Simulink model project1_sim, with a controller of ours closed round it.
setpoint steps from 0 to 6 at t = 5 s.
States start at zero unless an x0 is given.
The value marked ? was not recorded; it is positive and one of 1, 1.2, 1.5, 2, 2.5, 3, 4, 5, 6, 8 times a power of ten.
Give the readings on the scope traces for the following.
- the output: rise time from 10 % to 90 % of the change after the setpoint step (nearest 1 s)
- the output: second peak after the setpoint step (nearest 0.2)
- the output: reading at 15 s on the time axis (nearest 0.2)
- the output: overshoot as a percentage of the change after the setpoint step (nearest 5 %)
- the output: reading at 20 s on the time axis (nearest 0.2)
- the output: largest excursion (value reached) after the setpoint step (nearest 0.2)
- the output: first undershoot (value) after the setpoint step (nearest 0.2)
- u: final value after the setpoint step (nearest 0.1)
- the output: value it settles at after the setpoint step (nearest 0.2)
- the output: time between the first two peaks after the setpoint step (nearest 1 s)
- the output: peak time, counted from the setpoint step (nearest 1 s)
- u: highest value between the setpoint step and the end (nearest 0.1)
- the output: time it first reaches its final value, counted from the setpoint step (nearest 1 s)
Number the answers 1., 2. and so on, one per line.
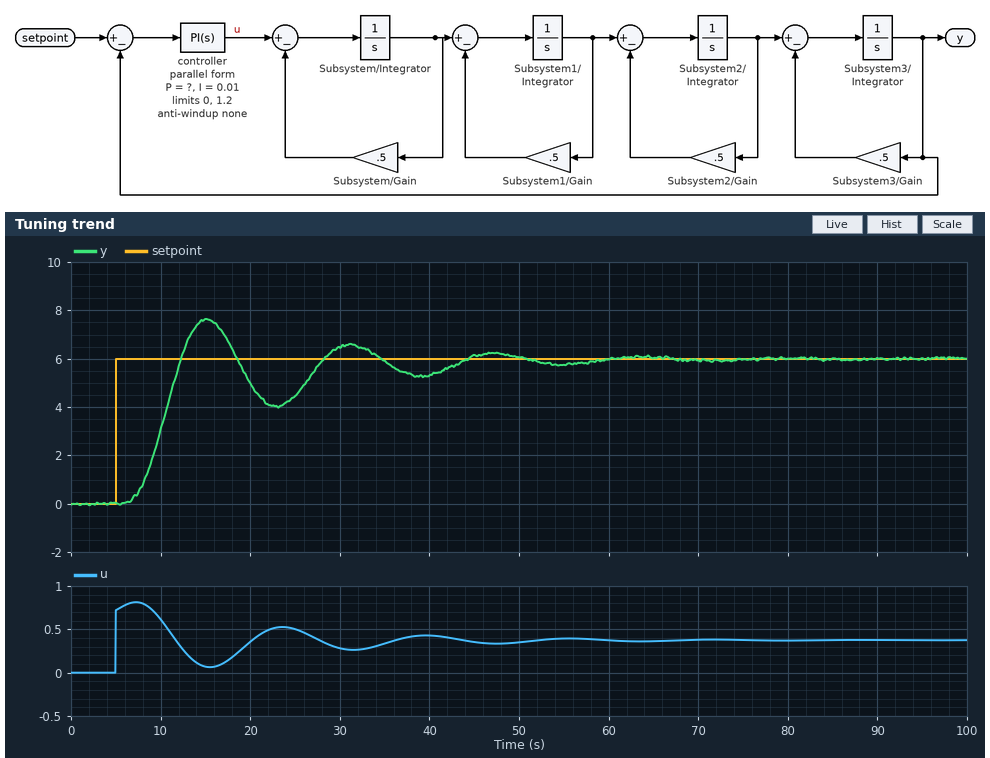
1. 4 s
2. 6.6
3. 7.6
4. 25 %
5. 5.0
6. 7.6
7. 4.0
8. 0.4
9. 6.0
10. 16 s
11. 10 s
12. 0.8
13. 7 s
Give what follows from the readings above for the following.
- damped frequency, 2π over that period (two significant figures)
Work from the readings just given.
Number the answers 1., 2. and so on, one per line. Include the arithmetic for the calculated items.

1. 2π / 16 = 0.39 rad/s
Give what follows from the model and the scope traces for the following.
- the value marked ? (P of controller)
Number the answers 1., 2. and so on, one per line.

1. 0.12
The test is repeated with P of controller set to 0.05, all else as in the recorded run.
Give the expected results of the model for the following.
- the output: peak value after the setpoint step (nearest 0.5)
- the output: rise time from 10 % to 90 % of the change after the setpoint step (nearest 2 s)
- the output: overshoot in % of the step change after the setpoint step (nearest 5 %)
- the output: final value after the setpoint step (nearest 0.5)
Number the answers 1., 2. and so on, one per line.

1. 7.0
2. 6 s
3. 15 %
4. 6.0
